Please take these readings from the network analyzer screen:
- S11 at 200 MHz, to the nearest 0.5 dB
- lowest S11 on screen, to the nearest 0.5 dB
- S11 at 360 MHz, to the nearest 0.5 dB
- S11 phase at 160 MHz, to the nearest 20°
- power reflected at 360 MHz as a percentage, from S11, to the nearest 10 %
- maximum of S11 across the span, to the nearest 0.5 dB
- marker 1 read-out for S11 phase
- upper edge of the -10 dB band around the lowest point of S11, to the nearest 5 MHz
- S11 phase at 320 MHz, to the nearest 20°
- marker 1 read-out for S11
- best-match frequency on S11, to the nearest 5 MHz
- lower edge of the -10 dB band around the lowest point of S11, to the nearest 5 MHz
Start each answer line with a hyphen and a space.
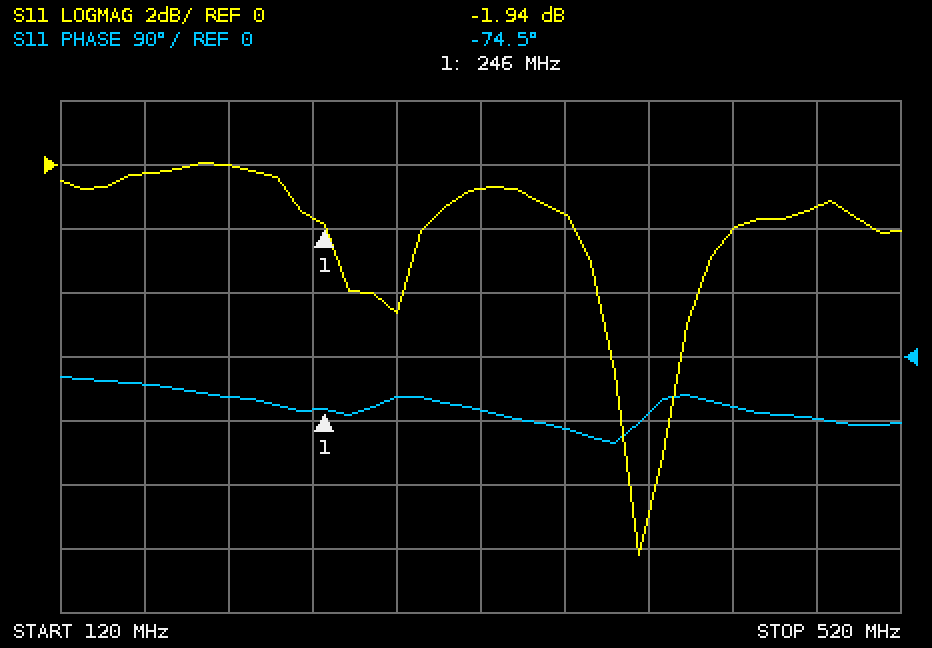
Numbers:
- 0.0 dB
- -12.0 dB
- -1.5 dB
- -40°
- 70 %
- 0.0 dB
- -74.5°
- 405 MHz
- -80°
- -1.94 dB
- 395 MHz
- 390 MHz
